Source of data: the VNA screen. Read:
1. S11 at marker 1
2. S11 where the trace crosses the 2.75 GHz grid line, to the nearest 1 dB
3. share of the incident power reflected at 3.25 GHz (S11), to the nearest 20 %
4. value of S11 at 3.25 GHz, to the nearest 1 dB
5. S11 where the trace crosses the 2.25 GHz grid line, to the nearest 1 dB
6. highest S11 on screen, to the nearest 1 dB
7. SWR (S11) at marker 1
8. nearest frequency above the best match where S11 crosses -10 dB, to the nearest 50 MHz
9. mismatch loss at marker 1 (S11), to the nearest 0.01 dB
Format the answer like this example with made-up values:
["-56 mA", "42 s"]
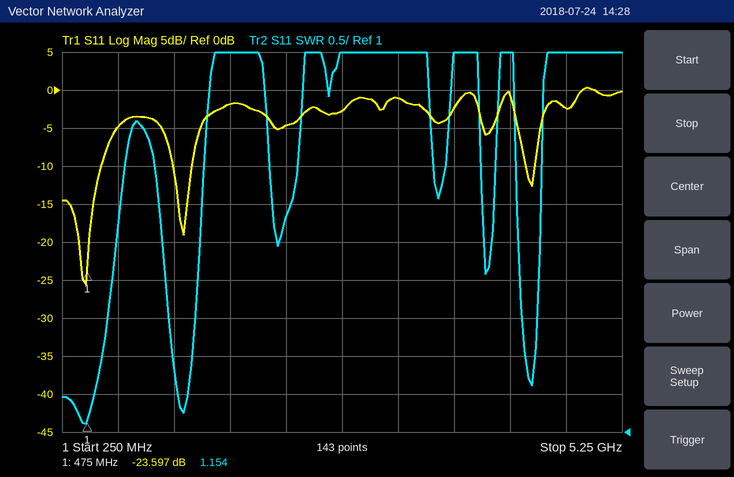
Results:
["-23.597 dB", "-3 dB", "80 %", "-1 dB", "-5 dB", "0 dB", "1.154", "600 MHz", "0.02 dB"]
